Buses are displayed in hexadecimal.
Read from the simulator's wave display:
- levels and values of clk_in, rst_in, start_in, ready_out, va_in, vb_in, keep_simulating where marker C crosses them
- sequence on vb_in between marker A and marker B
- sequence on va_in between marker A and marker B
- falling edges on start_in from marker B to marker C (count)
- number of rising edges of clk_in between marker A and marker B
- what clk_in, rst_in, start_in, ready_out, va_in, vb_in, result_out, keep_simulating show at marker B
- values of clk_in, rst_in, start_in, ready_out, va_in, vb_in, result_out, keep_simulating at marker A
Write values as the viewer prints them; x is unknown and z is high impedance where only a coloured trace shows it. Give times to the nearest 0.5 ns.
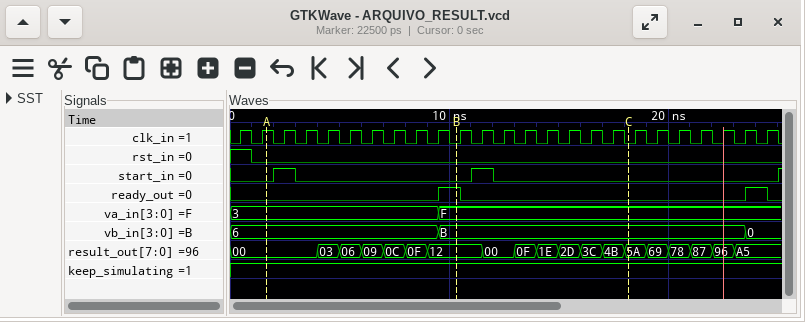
clk_in=0, rst_in=0, start_in=0, ready_out=0, va_in=F, vb_in=B, keep_simulating=1
6, B
3, F
1
8
clk_in=0, rst_in=0, start_in=0, ready_out=1, va_in=F, vb_in=B, result_out=12, keep_simulating=1
clk_in=1, rst_in=0, start_in=0, ready_out=0, va_in=3, vb_in=6, result_out=00, keep_simulating=1
